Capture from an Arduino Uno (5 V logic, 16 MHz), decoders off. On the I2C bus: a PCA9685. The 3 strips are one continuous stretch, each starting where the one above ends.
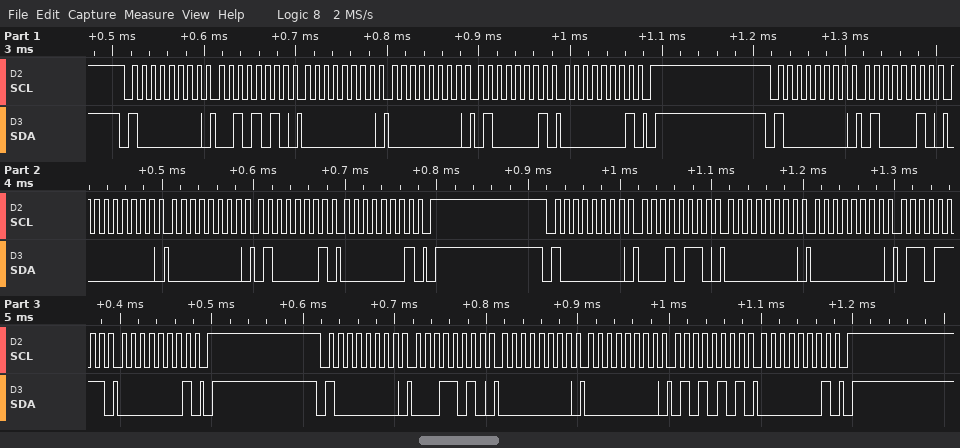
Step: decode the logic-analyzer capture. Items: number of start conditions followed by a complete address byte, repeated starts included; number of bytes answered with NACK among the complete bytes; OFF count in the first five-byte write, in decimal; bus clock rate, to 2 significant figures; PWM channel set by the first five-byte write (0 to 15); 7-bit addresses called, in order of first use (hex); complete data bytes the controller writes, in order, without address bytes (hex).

4
0
321
100 kHz
9
0x40
2A 00 00 41 01 42 00 00 41 01 16 00 00 6F 01 1A 00 00 55 01
